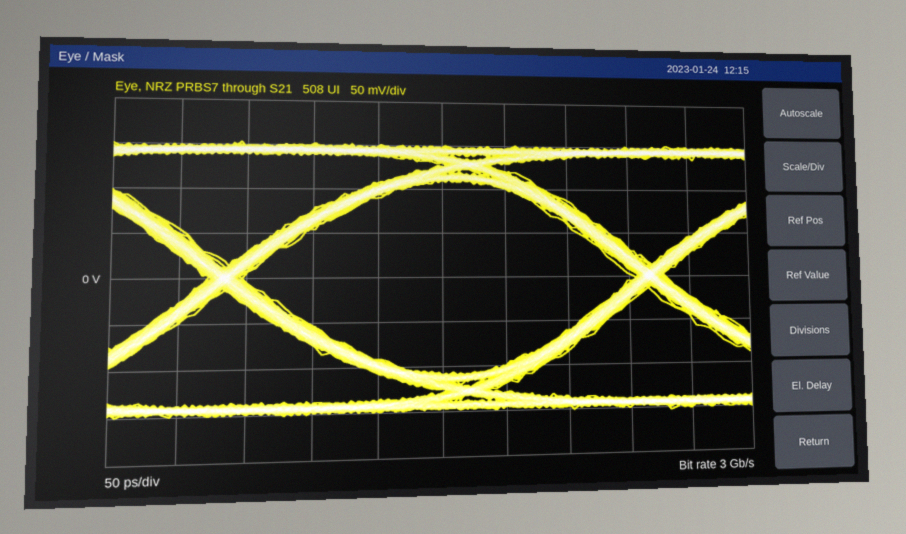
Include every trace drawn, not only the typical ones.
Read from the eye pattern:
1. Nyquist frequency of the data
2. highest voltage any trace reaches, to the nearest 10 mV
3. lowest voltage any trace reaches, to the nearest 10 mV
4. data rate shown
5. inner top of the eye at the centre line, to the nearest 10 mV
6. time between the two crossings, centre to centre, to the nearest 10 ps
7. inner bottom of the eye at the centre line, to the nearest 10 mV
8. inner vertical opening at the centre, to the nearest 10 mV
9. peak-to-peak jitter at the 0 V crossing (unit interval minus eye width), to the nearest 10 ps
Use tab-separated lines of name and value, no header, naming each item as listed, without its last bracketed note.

Nyquist frequency of the data	1.5 GHz
highest voltage any trace reaches, to the nearest 10 mV	150 mV
lowest voltage any trace reaches, to the nearest 10 mV	-150 mV
data rate shown	3 Gb/s
inner top of the eye at the centre line, to the nearest 10 mV	110 mV
time between the two crossings, centre to centre, to the nearest 10 ps	330 ps
inner bottom of the eye at the centre line, to the nearest 10 mV	-110 mV
inner vertical opening at the centre, to the nearest 10 mV	220 mV
peak-to-peak jitter at the 0 V crossing (unit interval minus eye width), to the nearest 10 ps	30 ps
